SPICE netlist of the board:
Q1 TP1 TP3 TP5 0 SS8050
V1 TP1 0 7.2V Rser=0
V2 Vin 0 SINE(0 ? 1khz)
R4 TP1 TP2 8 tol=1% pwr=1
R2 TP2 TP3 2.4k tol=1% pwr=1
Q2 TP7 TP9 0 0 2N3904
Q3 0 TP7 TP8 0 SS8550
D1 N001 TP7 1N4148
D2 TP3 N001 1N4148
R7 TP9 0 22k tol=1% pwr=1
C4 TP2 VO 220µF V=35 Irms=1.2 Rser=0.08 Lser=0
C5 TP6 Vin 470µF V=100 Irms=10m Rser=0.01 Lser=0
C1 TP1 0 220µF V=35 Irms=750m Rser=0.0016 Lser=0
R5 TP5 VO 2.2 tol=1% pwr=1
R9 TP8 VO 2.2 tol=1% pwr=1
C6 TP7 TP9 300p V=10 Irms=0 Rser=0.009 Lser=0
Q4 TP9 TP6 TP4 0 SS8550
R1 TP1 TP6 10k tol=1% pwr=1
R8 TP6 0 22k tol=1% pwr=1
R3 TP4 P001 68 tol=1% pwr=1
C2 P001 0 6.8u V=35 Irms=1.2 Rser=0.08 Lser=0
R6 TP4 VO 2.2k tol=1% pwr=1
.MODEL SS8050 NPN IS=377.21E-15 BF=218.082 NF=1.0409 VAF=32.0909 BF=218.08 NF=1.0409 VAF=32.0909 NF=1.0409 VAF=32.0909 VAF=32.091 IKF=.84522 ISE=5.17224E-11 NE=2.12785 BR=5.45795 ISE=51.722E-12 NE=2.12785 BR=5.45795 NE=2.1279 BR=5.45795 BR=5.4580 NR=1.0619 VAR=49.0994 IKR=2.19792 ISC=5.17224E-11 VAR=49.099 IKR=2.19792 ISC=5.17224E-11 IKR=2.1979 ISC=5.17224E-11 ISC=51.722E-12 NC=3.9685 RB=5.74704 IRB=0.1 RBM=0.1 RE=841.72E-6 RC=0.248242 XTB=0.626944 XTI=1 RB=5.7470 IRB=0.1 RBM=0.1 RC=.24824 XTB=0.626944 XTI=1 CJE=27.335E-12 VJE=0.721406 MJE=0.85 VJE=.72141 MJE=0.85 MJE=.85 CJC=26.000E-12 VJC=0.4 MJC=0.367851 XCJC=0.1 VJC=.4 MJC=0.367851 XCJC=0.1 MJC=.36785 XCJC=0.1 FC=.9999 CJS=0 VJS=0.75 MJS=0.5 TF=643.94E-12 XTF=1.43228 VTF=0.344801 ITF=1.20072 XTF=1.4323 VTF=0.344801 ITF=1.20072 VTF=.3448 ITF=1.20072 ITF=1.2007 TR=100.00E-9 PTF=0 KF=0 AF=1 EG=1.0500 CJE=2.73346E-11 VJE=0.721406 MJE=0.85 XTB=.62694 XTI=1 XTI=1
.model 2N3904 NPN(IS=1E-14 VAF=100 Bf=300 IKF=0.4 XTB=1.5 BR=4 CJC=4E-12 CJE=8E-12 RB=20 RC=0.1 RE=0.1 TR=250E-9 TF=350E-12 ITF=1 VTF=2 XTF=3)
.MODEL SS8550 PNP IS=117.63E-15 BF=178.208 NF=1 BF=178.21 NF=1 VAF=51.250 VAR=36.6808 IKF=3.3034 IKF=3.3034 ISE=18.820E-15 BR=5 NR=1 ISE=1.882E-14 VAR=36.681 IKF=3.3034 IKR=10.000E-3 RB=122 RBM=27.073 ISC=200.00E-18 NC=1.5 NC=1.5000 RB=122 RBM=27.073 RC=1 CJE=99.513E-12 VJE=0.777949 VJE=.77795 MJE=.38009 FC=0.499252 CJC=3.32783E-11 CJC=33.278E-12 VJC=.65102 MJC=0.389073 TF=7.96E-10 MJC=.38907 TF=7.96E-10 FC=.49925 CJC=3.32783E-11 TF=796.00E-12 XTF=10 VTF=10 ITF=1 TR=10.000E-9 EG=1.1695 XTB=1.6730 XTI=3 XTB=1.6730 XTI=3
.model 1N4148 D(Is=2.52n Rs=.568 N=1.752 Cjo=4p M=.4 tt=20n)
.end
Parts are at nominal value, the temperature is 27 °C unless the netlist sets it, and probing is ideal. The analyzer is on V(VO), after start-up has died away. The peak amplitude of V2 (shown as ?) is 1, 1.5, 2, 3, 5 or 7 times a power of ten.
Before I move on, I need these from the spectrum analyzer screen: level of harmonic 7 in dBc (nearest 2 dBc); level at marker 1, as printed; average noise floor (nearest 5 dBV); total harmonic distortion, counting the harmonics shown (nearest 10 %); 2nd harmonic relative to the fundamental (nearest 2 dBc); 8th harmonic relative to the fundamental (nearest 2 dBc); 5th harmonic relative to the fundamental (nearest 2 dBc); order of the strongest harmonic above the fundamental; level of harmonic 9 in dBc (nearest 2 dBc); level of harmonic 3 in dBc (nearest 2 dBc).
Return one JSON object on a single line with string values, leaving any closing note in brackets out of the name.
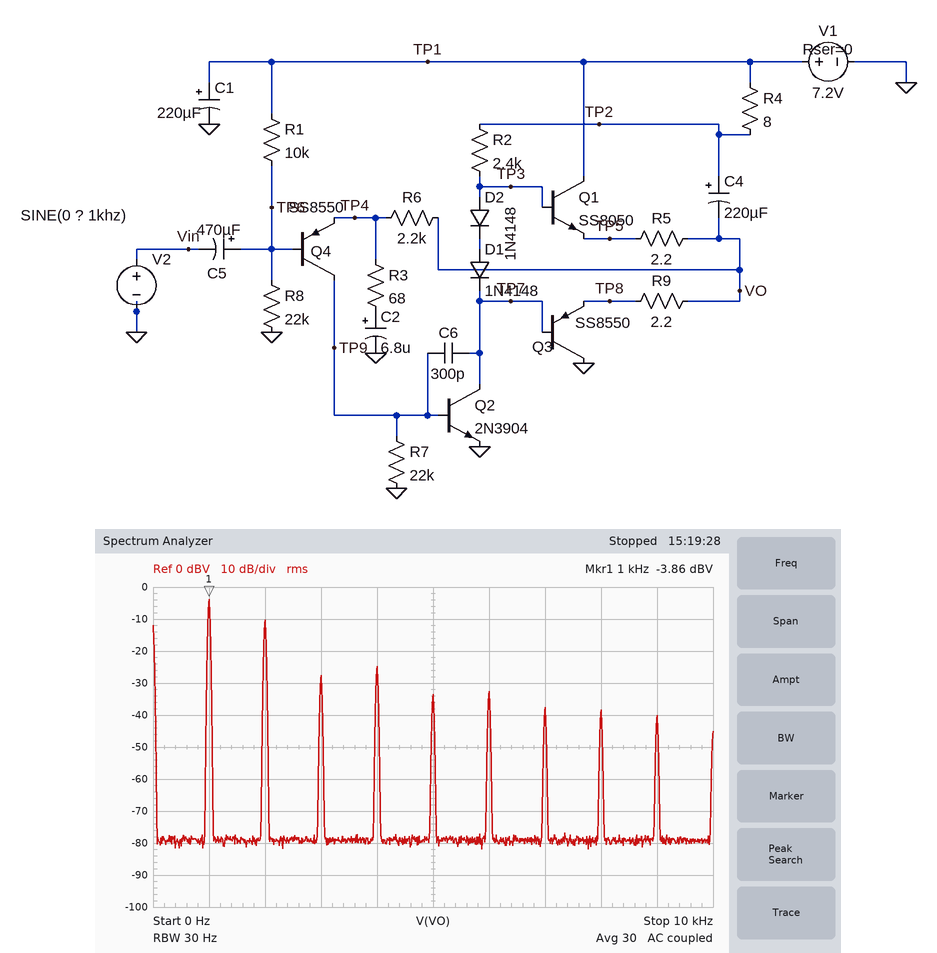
{"level of harmonic 7 in dBc": "-34 dBc", "level at marker 1, as printed": "-3.86 dBV", "average noise floor": "-80 dBV", "total harmonic distortion, counting the harmonics shown": "50 %", "2nd harmonic relative to the fundamental": "-6 dBc", "8th harmonic relative to the fundamental": "-34 dBc", "5th harmonic relative to the fundamental": "-30 dBc", "order of the strongest harmonic above the fundamental": "2", "level of harmonic 9 in dBc": "-36 dBc", "level of harmonic 3 in dBc": "-24 dBc"}
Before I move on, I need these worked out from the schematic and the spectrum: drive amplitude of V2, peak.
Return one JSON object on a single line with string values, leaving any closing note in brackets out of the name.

{"drive amplitude of V2, peak": "70 mV"}
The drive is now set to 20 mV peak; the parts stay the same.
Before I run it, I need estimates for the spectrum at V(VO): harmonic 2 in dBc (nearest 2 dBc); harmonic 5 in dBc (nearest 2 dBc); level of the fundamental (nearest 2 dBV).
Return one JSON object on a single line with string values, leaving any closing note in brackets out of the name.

{"harmonic 2 in dBc": "-28 dBc", "harmonic 5 in dBc": "-38 dBc", "level of the fundamental": "-8 dBV"}
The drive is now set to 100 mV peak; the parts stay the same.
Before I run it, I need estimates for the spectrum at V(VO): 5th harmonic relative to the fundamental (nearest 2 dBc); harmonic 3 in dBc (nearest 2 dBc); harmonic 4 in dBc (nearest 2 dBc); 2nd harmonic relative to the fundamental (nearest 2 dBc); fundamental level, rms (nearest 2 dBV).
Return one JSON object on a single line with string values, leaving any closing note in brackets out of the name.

{"5th harmonic relative to the fundamental": "-22 dBc", "harmonic 3 in dBc": "-16 dBc", "harmonic 4 in dBc": "-24 dBc", "2nd harmonic relative to the fundamental": "-4 dBc", "fundamental level, rms": "-4 dBV"}
